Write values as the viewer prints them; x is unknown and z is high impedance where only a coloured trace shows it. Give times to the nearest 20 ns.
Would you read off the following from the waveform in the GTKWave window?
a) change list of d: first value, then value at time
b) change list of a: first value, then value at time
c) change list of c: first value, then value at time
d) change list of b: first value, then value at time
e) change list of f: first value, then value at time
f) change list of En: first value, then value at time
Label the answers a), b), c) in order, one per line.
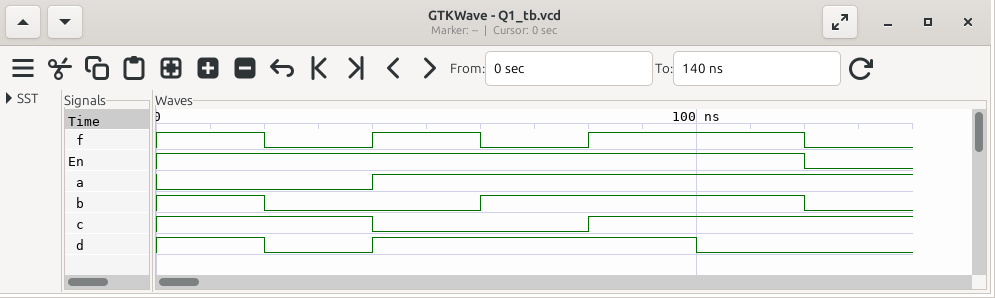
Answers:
a) 1, 0 at 20 ns, 1 at 40 ns, 0 at 100 ns
b) 0, 1 at 40 ns
c) 1, 0 at 40 ns, 1 at 80 ns
d) 1, 0 at 20 ns, 1 at 60 ns, 0 at 120 ns
e) 1, 0 at 20 ns, 1 at 40 ns, 0 at 60 ns, 1 at 80 ns, 0 at 120 ns
f) 1, 0 at 120 ns
